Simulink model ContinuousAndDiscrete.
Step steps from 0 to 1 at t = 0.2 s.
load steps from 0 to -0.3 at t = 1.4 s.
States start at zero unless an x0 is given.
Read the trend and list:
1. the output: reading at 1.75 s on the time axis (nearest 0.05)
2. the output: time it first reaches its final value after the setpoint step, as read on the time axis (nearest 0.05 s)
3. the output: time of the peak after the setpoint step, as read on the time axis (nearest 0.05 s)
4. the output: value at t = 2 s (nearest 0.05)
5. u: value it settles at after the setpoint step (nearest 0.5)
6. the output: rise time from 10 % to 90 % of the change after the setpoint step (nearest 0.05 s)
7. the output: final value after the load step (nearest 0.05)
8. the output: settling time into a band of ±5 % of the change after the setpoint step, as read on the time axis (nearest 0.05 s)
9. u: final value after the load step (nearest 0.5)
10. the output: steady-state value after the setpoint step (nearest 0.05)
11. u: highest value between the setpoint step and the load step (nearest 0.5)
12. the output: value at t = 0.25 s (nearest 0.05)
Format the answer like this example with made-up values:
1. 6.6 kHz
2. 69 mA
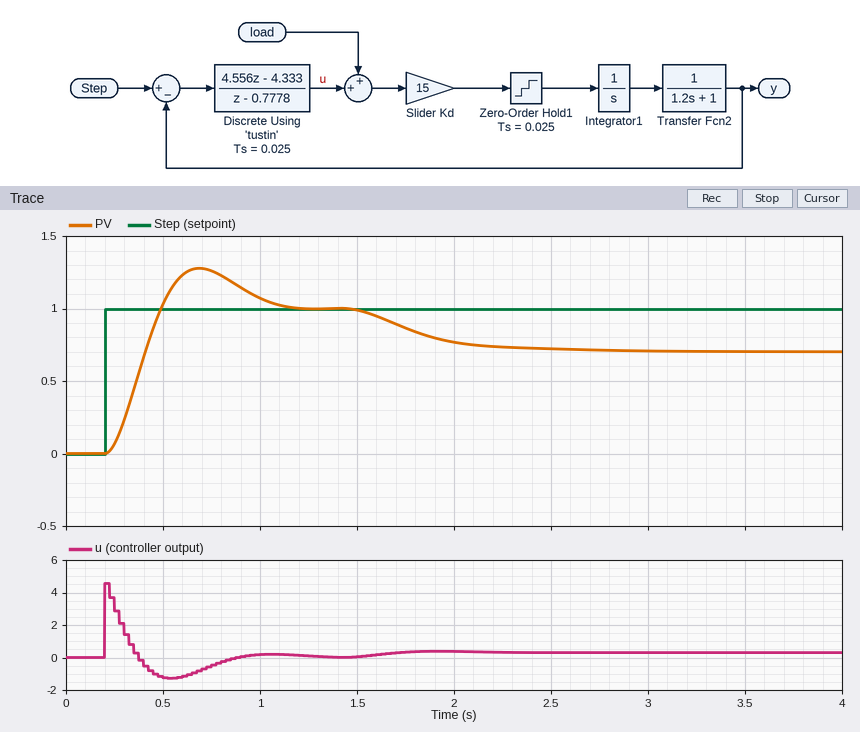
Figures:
1. 0.85
2. 0.50 s
3. 0.70 s
4. 0.75
5. 0.0
6. 0.20 s
7. 0.70
8. 1.05 s
9. 0.5
10. 1.00
11. 4.5
12. 0.05
